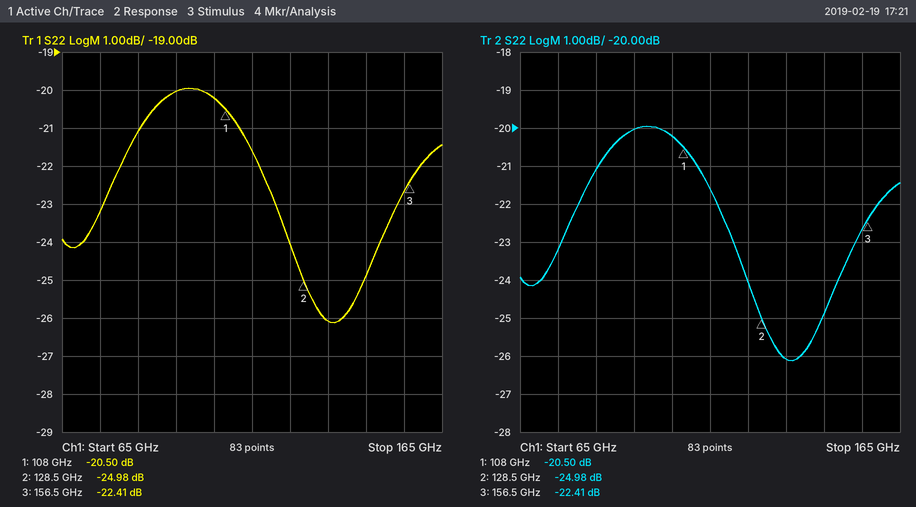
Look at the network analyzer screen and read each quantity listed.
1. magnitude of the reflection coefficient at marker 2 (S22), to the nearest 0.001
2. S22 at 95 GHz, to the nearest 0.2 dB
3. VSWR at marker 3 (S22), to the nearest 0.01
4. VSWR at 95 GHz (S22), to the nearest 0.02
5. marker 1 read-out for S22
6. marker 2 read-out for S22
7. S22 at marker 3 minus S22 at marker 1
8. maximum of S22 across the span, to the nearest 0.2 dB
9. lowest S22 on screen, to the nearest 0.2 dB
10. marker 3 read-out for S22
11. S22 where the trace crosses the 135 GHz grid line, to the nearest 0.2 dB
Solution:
0.056
-20.0 dB
1.16
1.22
-20.50 dB
-24.98 dB
-1.91 dB
-20.0 dB
-26.2 dB
-22.41 dB
-26.0 dB
